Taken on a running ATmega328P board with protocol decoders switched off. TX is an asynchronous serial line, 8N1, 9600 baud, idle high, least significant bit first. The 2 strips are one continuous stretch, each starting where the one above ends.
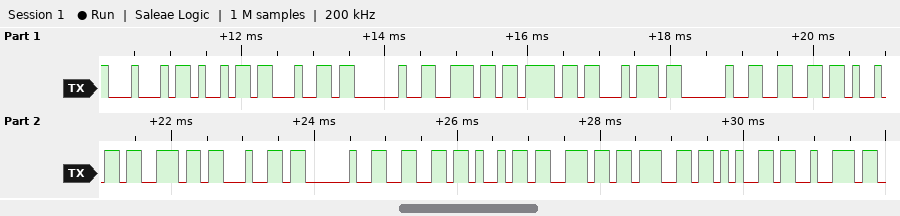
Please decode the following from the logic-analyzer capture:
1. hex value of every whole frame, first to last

44 69 64 20 6E 6F 74 20 66 69 6E 64 20 66 69 6E 67 65 72
